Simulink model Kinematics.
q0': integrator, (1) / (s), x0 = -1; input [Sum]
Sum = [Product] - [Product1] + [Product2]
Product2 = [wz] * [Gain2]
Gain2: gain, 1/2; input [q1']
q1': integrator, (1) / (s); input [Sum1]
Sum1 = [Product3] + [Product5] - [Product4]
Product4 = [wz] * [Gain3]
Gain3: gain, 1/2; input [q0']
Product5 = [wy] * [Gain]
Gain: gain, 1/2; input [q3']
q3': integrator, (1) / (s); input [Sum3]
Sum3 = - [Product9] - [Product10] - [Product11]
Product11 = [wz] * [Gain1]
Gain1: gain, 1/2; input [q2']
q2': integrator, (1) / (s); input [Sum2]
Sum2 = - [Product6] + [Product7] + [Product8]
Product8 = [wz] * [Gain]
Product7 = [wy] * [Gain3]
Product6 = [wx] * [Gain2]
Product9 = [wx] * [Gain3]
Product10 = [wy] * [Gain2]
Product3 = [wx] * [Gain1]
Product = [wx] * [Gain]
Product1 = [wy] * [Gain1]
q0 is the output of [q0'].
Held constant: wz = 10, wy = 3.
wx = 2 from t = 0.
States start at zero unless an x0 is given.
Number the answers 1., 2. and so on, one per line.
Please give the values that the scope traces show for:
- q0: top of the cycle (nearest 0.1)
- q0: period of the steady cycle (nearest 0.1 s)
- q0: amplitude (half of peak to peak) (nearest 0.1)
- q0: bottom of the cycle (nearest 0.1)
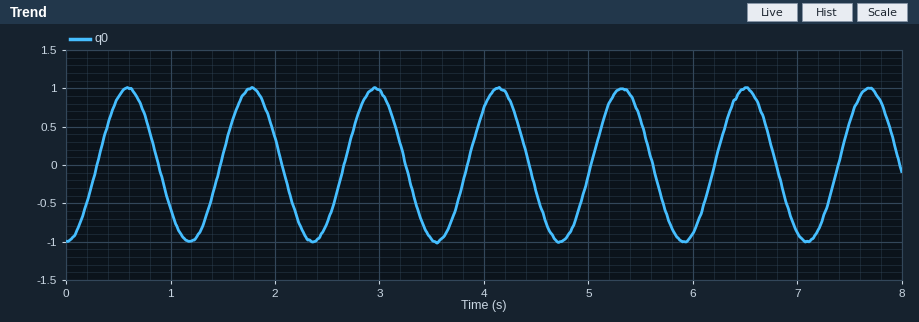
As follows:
1. 1.0
2. 1.2 s
3. 1.0
4. -1.0
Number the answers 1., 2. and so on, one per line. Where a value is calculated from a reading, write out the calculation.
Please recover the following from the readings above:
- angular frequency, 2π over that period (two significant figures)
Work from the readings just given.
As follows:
1. 2π / 1.2 = 5.2 rad/s
